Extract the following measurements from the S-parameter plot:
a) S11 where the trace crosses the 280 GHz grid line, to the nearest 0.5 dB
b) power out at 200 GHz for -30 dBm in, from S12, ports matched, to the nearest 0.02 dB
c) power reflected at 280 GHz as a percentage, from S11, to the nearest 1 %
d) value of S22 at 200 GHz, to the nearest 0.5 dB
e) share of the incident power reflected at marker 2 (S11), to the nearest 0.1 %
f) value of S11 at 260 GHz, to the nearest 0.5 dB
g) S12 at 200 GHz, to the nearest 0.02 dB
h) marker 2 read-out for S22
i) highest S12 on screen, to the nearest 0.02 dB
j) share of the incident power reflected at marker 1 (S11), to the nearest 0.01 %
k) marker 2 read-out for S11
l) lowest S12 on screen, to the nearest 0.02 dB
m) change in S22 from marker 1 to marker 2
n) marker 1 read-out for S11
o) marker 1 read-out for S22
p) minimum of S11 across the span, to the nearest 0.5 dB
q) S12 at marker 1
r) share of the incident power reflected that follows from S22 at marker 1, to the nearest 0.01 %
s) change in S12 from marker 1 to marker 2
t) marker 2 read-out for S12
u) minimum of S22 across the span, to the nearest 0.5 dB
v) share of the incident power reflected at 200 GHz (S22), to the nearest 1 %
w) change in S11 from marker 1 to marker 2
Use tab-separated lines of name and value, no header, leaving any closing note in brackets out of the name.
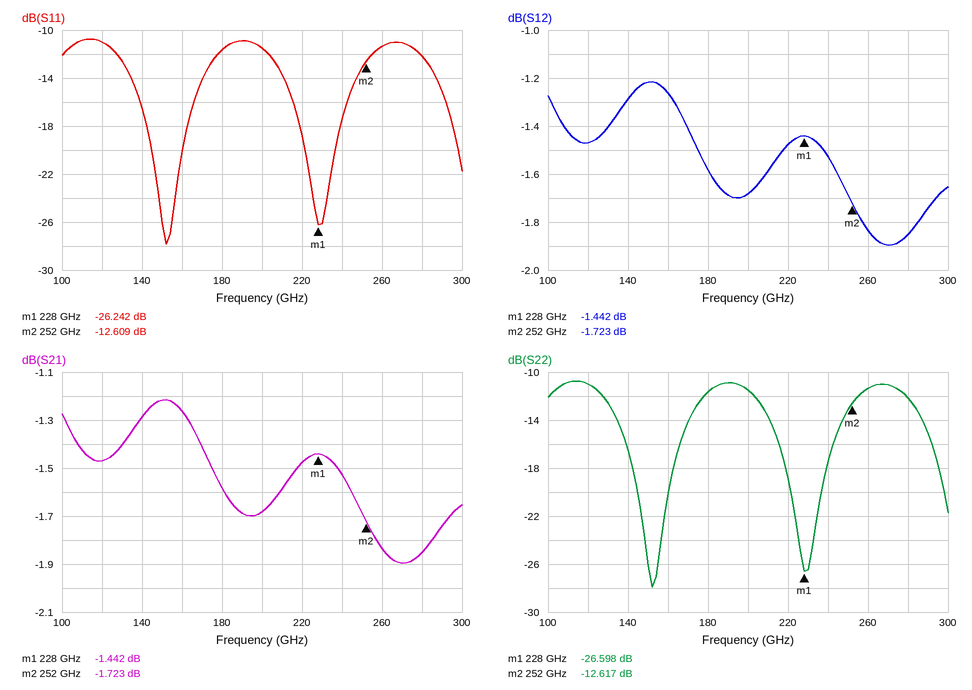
S11 where the trace crosses the 280 GHz grid line, to the nearest 0.5 dB	-12.0 dB
power out at 200 GHz for -30 dBm in, from S12, ports matched, to the nearest 0.02 dB	-31.68 dBm
power reflected at 280 GHz as a percentage, from S11, to the nearest 1 %	6 %
value of S22 at 200 GHz, to the nearest 0.5 dB	-11.5 dB
share of the incident power reflected at marker 2 (S11), to the nearest 0.1 %	5.5 %
value of S11 at 260 GHz, to the nearest 0.5 dB	-11.5 dB
S12 at 200 GHz, to the nearest 0.02 dB	-1.68 dB
marker 2 read-out for S22	-12.617 dB
highest S12 on screen, to the nearest 0.02 dB	-1.22 dB
share of the incident power reflected at marker 1 (S11), to the nearest 0.01 %	0.24 %
marker 2 read-out for S11	-12.609 dB
lowest S12 on screen, to the nearest 0.02 dB	-1.90 dB
change in S22 from marker 1 to marker 2	13.981 dB
marker 1 read-out for S11	-26.242 dB
marker 1 read-out for S22	-26.598 dB
minimum of S11 across the span, to the nearest 0.5 dB	-28.0 dB
S12 at marker 1	-1.442 dB
share of the incident power reflected that follows from S22 at marker 1, to the nearest 0.01 %	0.22 %
change in S12 from marker 1 to marker 2	-0.281 dB
marker 2 read-out for S12	-1.723 dB
minimum of S22 across the span, to the nearest 0.5 dB	-28.0 dB
share of the incident power reflected at 200 GHz (S22), to the nearest 1 %	7 %
change in S11 from marker 1 to marker 2	13.633 dB
